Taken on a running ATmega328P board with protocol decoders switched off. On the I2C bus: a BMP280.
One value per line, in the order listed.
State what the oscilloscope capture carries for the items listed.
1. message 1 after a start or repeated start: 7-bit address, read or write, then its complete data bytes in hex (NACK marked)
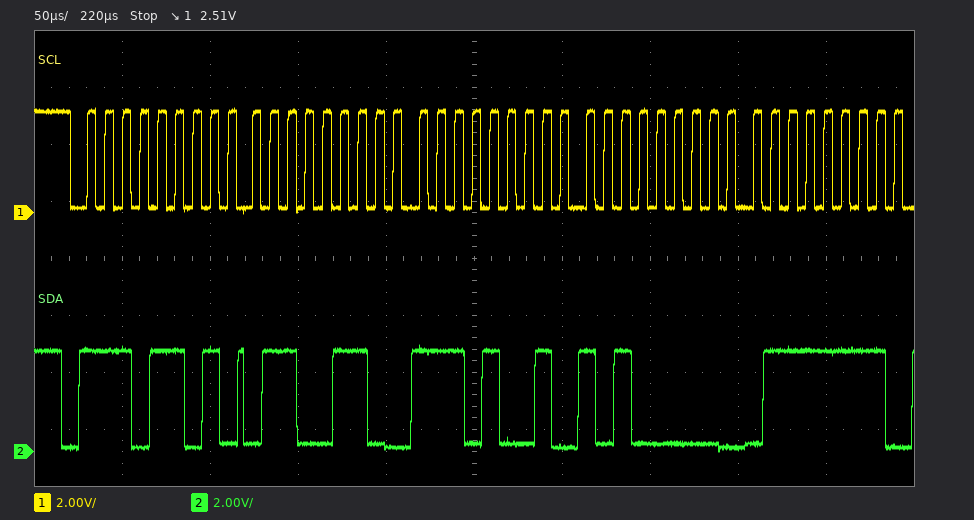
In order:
0x76 read: 66 E9 A0 7F
